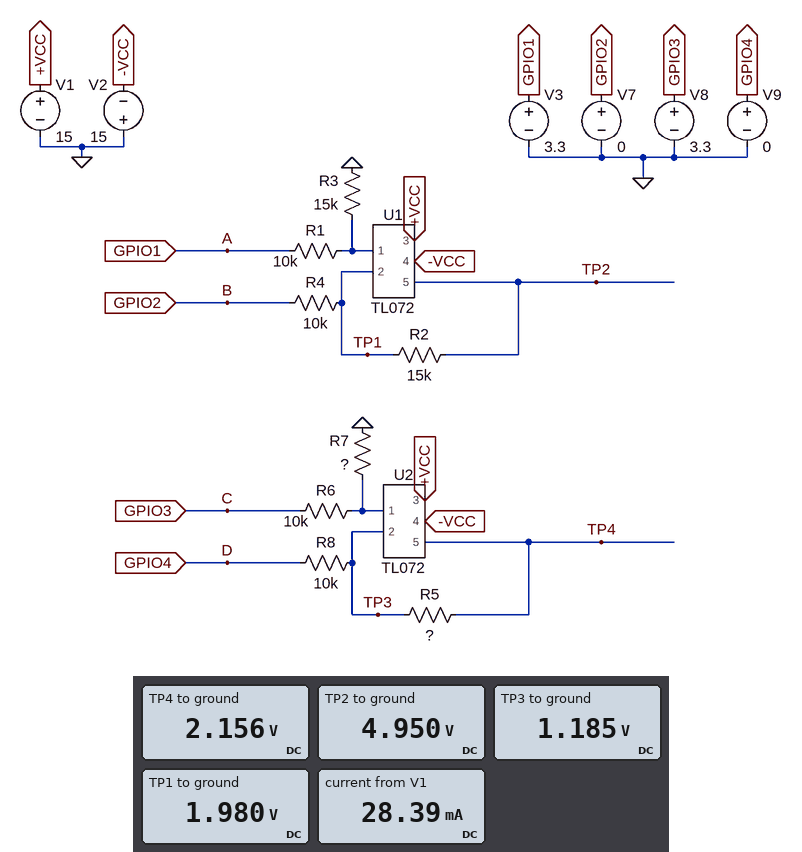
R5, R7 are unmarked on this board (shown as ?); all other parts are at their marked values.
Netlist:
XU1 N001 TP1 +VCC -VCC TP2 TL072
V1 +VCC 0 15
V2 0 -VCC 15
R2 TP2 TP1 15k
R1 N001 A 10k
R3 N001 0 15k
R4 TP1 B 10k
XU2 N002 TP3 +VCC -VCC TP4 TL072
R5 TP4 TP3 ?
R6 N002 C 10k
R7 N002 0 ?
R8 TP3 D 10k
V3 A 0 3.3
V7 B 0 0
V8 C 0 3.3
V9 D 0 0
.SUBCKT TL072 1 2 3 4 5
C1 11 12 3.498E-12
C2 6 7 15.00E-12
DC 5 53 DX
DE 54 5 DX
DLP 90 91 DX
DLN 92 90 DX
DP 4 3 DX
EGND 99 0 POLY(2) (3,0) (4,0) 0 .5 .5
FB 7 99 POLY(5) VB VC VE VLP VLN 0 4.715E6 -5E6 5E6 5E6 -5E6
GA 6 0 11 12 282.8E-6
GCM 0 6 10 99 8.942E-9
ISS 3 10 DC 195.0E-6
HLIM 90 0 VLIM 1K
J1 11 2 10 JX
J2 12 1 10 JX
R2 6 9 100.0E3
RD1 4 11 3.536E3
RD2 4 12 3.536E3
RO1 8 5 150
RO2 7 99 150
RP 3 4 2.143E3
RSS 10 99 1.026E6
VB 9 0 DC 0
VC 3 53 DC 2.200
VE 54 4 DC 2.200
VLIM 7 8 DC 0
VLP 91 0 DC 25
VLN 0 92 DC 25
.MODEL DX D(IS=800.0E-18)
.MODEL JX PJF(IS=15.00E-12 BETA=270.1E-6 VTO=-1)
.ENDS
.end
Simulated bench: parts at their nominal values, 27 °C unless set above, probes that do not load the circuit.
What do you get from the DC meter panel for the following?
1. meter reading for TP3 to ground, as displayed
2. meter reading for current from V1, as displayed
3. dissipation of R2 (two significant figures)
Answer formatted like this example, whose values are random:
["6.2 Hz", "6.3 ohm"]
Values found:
["1.185 V", "28.39 mA", "590 µW"]
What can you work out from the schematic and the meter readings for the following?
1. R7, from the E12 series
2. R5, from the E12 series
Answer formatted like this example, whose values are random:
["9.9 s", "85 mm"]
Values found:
["5.6 kΩ", "8.2 kΩ"]
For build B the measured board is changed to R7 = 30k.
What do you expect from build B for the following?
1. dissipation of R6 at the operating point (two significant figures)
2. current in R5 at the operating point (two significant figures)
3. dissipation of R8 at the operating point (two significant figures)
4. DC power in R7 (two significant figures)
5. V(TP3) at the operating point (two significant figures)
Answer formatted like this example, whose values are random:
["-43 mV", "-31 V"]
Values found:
["68 µW", "250 µA", "610 µW", "200 µW", "2.5 V"]
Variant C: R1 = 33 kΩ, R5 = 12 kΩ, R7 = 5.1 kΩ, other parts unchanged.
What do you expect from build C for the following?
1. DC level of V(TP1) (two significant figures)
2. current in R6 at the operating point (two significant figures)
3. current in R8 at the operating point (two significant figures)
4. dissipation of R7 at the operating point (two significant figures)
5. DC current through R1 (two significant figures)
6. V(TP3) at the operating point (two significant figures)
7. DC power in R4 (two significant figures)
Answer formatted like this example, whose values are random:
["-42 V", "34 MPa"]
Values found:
["1.0 V", "220 µA", "110 µA", "240 µW", "69 µA", "1.1 V", "110 µW"]
